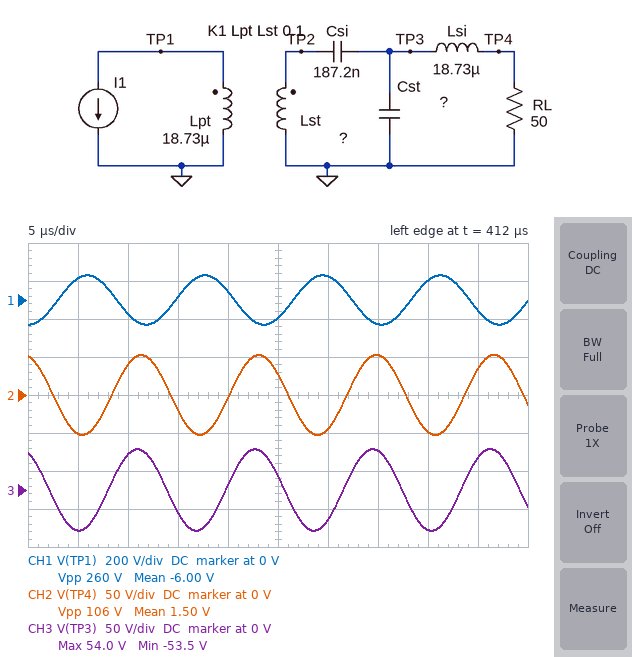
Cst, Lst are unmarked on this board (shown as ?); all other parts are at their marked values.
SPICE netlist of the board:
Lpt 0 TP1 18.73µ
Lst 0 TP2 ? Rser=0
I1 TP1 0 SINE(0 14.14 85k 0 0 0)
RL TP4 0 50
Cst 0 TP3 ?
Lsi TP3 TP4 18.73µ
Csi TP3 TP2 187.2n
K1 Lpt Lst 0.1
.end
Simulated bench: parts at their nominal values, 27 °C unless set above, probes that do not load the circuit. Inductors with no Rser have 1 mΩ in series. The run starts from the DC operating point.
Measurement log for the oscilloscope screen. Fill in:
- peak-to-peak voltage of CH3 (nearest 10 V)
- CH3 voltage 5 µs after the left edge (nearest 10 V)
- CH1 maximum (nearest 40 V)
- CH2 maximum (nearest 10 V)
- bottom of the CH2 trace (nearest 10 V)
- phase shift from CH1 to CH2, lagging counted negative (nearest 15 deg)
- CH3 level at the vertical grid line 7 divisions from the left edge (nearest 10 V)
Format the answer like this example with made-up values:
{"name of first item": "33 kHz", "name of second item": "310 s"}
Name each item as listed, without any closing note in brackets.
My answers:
{"peak-to-peak voltage of CH3": "110 V", "CH3 voltage 5 µs after the left edge": "-50 V", "CH1 maximum": "120 V", "CH2 maximum": "50 V", "bottom of the CH2 trace": "-50 V", "phase shift from CH1 to CH2, lagging counted negative": "-165 deg", "CH3 level at the vertical grid line 7 divisions from the left edge": "50 V"}
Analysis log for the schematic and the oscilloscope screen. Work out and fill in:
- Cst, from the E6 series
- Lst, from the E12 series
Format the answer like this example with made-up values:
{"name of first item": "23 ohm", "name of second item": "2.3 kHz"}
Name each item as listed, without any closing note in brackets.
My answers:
{"Cst, from the E6 series": "330 nF", "Lst, from the E12 series": "33 µH"}
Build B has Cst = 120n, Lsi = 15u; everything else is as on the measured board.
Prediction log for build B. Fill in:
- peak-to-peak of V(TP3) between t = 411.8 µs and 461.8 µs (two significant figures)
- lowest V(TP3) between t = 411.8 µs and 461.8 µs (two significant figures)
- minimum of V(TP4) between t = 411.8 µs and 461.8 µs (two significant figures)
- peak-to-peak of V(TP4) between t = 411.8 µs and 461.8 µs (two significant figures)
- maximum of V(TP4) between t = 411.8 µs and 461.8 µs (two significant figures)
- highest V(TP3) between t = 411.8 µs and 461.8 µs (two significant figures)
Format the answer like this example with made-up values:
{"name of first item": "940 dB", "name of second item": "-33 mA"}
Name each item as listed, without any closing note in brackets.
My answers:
{"peak-to-peak of V(TP3) between t = 411.8 µs and 461.8 µs": "68 V", "lowest V(TP3) between t = 411.8 µs and 461.8 µs": "-34 V", "minimum of V(TP4) between t = 411.8 µs and 461.8 µs": "-33 V", "peak-to-peak of V(TP4) between t = 411.8 µs and 461.8 µs": "67 V", "maximum of V(TP4) between t = 411.8 µs and 461.8 µs": "33 V", "highest V(TP3) between t = 411.8 µs and 461.8 µs": "34 V"}
